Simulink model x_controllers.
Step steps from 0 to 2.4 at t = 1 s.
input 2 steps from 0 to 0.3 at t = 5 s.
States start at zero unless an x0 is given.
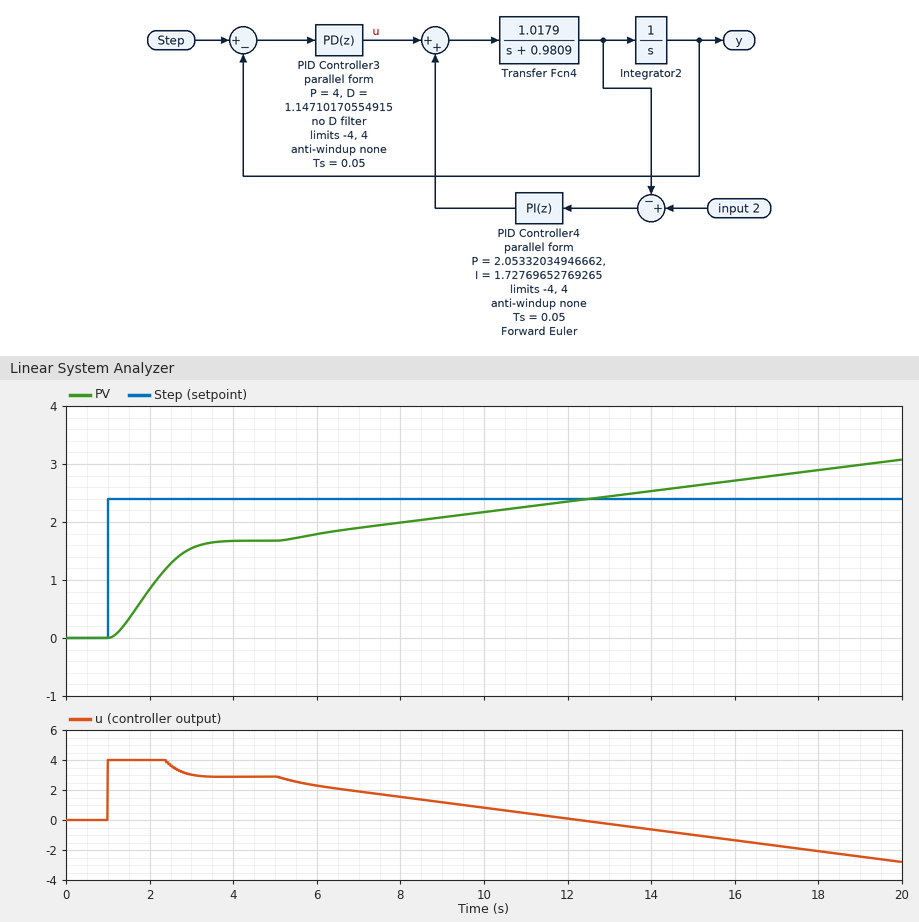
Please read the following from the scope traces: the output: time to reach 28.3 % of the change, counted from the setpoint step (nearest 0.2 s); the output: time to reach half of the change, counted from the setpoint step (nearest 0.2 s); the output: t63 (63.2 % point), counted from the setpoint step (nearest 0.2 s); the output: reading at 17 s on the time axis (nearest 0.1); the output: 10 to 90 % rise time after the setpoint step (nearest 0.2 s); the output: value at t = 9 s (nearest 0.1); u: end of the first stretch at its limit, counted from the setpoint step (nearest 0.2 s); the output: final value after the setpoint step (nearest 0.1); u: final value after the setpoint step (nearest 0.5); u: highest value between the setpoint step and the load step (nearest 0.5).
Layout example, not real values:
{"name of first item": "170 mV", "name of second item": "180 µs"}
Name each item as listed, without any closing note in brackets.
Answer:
{"the output: time to reach 28.3 % of the change, counted from the setpoint step": "0.6 s", "the output: time to reach half of the change, counted from the setpoint step": "1.0 s", "the output: t63 (63.2 % point), counted from the setpoint step": "1.2 s", "the output: reading at 17 s on the time axis": "2.8", "the output: 10 to 90 % rise time after the setpoint step": "1.6 s", "the output: value at t = 9 s": "2.1", "u: end of the first stretch at its limit, counted from the setpoint step": "1.4 s", "the output: final value after the setpoint step": "1.7", "u: final value after the setpoint step": "3.0", "u: highest value between the setpoint step and the load step": "4.0"}
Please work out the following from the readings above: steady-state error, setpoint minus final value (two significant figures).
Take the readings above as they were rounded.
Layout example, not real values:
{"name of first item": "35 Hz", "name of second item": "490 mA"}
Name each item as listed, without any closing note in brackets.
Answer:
{"steady-state error, setpoint minus final value": "0.70"}
